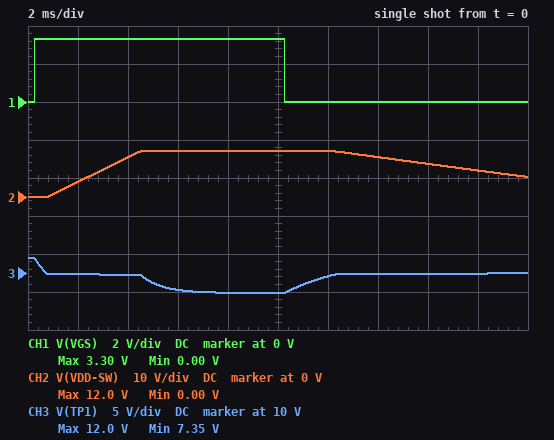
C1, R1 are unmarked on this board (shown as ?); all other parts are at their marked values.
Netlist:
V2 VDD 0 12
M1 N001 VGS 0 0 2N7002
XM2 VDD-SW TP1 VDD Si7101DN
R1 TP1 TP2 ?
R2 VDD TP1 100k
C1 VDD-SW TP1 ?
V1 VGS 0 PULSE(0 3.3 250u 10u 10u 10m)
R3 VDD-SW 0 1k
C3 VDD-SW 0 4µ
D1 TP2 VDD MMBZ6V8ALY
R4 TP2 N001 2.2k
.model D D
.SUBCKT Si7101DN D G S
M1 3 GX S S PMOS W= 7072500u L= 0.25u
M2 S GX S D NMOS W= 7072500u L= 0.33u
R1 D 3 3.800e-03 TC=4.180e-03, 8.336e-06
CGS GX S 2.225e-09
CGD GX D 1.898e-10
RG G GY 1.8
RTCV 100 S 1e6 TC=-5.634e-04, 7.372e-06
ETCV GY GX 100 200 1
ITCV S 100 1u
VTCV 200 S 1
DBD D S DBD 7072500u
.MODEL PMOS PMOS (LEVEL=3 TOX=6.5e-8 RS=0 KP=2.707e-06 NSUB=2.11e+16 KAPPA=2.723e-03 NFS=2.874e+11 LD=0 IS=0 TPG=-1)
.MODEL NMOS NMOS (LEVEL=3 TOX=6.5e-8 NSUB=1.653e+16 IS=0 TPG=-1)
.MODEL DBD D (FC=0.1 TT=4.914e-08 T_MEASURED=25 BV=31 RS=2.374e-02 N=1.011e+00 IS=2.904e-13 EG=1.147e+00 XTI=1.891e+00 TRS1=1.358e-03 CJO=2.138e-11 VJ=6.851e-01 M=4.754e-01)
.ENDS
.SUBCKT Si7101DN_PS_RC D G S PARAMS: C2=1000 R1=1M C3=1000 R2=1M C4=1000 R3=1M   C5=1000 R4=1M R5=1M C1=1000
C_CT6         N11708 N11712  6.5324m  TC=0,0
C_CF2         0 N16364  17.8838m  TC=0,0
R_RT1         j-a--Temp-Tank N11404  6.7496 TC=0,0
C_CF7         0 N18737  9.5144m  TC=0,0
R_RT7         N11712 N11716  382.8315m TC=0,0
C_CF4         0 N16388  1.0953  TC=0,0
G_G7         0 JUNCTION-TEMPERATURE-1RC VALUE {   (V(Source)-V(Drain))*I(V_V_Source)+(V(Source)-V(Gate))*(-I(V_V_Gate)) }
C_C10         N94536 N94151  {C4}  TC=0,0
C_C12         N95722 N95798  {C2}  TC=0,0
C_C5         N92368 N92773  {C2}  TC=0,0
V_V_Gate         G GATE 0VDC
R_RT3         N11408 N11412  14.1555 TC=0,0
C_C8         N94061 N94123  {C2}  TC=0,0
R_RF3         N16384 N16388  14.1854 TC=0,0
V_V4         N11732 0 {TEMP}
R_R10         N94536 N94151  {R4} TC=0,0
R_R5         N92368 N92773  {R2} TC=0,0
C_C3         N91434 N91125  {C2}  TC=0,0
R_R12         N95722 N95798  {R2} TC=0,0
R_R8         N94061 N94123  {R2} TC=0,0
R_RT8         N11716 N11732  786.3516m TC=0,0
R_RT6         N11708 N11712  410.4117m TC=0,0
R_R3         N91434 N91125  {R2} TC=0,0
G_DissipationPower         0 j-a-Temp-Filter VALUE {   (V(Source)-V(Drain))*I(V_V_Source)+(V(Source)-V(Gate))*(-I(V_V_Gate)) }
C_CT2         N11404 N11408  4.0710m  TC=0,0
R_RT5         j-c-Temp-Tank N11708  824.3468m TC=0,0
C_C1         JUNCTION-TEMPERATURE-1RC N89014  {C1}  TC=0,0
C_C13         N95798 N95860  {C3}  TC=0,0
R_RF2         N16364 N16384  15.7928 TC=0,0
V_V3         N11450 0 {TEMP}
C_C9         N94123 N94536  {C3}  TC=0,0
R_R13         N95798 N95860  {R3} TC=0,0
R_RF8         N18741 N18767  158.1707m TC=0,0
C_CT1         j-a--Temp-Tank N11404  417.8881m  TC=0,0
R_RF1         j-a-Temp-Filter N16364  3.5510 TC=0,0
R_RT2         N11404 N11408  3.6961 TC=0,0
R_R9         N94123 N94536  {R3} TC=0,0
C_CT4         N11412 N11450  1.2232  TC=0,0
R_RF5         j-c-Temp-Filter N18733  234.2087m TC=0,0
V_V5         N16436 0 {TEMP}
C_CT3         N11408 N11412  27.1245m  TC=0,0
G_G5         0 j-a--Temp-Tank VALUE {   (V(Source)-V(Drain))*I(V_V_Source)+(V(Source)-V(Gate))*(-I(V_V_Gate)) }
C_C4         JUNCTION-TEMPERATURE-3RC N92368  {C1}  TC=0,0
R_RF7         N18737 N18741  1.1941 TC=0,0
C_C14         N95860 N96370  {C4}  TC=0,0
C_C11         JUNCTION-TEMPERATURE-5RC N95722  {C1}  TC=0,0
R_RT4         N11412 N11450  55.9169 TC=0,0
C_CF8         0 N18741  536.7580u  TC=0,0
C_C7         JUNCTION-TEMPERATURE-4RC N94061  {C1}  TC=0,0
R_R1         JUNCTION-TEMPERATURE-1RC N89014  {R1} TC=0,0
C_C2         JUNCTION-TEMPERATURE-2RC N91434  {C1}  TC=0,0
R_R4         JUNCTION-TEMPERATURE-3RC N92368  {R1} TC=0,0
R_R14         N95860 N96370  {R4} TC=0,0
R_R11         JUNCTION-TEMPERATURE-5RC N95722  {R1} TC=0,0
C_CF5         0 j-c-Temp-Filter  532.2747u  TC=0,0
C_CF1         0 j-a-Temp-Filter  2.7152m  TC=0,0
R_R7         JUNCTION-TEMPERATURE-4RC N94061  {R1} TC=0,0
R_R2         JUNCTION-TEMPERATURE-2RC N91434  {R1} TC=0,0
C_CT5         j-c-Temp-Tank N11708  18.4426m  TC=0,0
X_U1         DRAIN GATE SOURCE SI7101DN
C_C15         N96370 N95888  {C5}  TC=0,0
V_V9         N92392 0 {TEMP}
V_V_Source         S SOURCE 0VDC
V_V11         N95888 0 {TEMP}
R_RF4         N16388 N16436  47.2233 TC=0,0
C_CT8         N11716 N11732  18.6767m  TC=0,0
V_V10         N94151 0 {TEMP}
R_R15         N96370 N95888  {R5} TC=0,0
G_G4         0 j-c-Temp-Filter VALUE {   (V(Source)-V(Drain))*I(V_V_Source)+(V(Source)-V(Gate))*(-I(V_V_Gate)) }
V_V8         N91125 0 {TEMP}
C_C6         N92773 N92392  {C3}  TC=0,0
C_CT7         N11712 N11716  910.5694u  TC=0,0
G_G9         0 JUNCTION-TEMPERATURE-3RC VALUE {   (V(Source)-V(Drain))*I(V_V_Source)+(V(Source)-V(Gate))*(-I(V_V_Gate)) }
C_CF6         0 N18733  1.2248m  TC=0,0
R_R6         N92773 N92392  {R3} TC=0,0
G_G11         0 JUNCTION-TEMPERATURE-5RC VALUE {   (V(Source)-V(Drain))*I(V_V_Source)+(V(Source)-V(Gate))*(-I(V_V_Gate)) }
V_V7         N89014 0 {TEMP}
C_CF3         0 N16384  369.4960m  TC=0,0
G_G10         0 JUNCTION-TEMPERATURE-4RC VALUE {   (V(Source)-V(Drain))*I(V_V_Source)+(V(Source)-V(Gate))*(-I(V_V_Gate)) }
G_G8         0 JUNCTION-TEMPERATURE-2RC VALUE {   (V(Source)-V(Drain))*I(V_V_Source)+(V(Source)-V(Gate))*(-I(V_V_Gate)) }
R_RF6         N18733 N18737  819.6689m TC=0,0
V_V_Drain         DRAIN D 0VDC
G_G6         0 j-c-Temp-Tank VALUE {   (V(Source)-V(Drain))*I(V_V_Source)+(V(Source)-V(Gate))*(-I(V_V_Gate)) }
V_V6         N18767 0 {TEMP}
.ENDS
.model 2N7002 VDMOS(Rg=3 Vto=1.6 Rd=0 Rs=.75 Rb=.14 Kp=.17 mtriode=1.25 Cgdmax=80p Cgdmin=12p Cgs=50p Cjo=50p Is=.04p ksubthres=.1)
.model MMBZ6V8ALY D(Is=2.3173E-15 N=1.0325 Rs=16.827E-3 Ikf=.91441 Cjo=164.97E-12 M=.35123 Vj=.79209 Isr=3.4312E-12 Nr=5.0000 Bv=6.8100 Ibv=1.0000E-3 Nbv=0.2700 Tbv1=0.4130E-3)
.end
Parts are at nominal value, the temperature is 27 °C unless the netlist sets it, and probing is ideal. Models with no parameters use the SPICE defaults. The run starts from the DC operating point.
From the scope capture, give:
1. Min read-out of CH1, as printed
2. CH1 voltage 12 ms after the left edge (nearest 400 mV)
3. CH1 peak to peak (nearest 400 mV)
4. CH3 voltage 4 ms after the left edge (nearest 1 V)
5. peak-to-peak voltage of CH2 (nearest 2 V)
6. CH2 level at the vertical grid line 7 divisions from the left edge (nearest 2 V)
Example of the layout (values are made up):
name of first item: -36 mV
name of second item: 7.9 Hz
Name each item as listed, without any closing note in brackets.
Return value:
Min read-out of CH1, as printed: 0.00 V
CH1 voltage 12 ms after the left edge: 0 V
CH1 peak to peak: 3.2 V
CH3 voltage 4 ms after the left edge: 10 V
peak-to-peak voltage of CH2: 12 V
CH2 level at the vertical grid line 7 divisions from the left edge: 10 V
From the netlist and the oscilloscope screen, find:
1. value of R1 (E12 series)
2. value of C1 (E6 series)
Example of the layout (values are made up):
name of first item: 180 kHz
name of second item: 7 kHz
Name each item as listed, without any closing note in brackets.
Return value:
value of R1: 47 kΩ
value of C1: 22 nF
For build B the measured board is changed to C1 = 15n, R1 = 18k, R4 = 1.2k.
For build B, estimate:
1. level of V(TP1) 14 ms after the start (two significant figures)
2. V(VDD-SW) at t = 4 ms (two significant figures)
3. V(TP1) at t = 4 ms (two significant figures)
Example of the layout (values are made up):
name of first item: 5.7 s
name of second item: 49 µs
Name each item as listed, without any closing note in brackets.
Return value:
level of V(TP1) 14 ms after the start: 9.9 V
V(VDD-SW) at t = 4 ms: 12 V
V(TP1) at t = 4 ms: 6.2 V
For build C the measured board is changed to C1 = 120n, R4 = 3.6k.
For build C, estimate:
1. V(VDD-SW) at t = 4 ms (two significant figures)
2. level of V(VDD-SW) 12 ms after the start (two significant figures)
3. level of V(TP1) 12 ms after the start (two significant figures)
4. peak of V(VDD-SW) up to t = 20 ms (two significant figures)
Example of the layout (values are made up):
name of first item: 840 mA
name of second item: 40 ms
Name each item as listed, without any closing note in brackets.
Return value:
V(VDD-SW) at t = 4 ms: 910 mV
level of V(VDD-SW) 12 ms after the start: 4.7 V
level of V(TP1) 12 ms after the start: 9.9 V
peak of V(VDD-SW) up to t = 20 ms: 5.0 V
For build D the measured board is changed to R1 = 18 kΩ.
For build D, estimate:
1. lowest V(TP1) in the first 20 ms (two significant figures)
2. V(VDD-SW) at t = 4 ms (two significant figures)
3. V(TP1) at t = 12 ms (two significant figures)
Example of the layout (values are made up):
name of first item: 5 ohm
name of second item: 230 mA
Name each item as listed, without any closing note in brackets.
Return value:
lowest V(TP1) in the first 20 ms: 6.2 V
V(VDD-SW) at t = 4 ms: 12 V
V(TP1) at t = 12 ms: 9.0 V
